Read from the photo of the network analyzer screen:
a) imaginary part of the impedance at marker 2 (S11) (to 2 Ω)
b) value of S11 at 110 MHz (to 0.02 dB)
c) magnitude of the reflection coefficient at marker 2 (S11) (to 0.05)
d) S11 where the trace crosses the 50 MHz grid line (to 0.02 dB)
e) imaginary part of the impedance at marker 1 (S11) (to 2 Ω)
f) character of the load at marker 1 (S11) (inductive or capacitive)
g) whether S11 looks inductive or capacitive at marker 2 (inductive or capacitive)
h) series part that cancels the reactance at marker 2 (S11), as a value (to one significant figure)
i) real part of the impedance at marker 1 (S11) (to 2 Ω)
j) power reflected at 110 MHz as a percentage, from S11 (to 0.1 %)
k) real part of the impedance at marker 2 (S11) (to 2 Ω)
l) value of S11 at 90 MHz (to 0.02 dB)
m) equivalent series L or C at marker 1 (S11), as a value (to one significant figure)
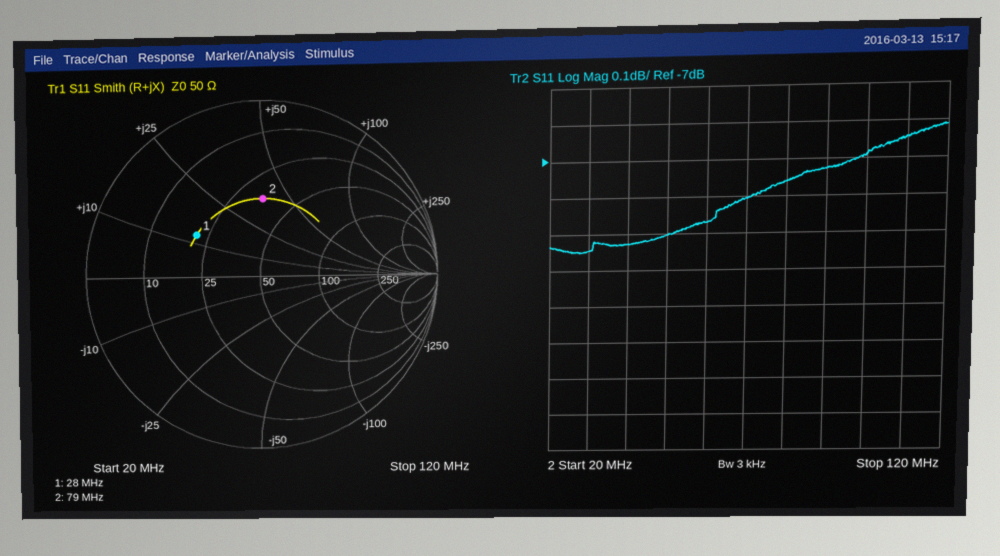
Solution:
+38 Ω
-6.94 dB
0.45
-7.20 dB
+12 Ω
inductive
inductive
50 pF
22 Ω
20.2 %
34 Ω
-7.02 dB
70 nH
